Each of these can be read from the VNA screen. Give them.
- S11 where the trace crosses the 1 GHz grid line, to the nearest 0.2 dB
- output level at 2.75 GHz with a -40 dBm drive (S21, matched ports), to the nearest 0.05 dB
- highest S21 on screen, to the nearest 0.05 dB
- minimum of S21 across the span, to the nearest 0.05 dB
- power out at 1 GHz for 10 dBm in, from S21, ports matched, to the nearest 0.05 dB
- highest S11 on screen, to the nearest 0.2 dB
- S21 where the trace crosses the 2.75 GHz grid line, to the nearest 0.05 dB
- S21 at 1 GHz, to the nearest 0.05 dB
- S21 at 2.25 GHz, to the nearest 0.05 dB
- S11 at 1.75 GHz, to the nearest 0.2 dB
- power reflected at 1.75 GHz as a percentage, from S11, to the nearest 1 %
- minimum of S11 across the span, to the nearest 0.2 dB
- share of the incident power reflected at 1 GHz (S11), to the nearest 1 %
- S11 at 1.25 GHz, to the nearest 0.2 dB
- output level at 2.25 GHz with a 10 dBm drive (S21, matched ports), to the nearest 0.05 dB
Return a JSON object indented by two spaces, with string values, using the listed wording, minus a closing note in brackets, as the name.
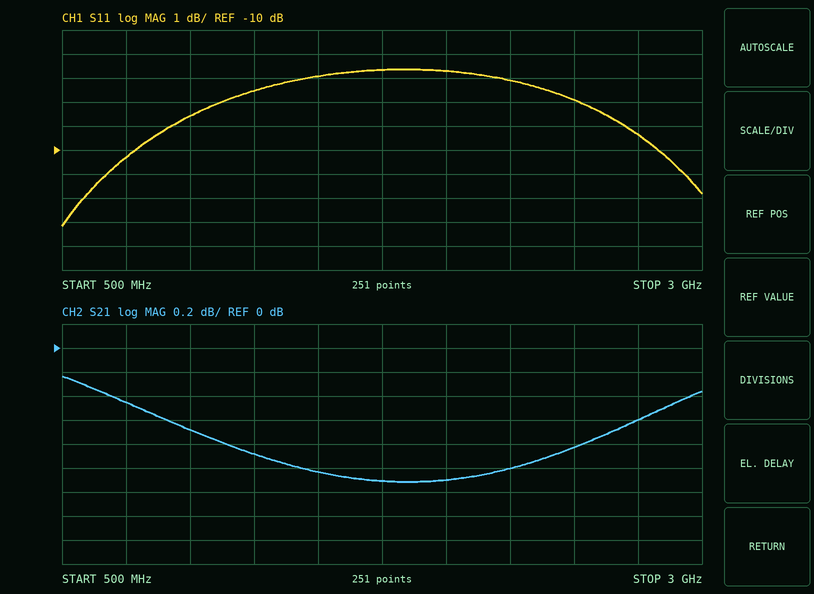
{
  "S11 where the trace crosses the 1 GHz grid line, to the nearest 0.2 dB": "-8.6 dB",
  "output level at 2.75 GHz with a -40 dBm drive (S21, matched ports), to the nearest 0.05 dB": "-40.60 dBm",
  "highest S21 on screen, to the nearest 0.05 dB": "-0.25 dB",
  "minimum of S21 across the span, to the nearest 0.05 dB": "-1.10 dB",
  "power out at 1 GHz for 10 dBm in, from S21, ports matched, to the nearest 0.05 dB": "9.30 dBm",
  "highest S11 on screen, to the nearest 0.2 dB": "-6.6 dB",
  "S21 where the trace crosses the 2.75 GHz grid line, to the nearest 0.05 dB": "-0.60 dB",
  "S21 at 1 GHz, to the nearest 0.05 dB": "-0.70 dB",
  "S21 at 2.25 GHz, to the nearest 0.05 dB": "-1.00 dB",
  "S11 at 1.75 GHz, to the nearest 0.2 dB": "-6.6 dB",
  "power reflected at 1.75 GHz as a percentage, from S11, to the nearest 1 %": "22 %",
  "minimum of S11 across the span, to the nearest 0.2 dB": "-13.2 dB",
  "share of the incident power reflected at 1 GHz (S11), to the nearest 1 %": "14 %",
  "S11 at 1.25 GHz, to the nearest 0.2 dB": "-7.6 dB",
  "output level at 2.25 GHz with a 10 dBm drive (S21, matched ports), to the nearest 0.05 dB": "9.00 dBm"
}
